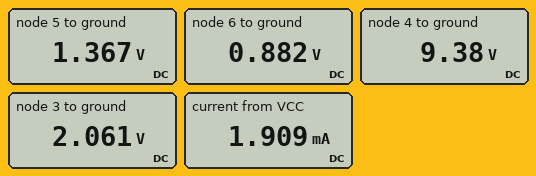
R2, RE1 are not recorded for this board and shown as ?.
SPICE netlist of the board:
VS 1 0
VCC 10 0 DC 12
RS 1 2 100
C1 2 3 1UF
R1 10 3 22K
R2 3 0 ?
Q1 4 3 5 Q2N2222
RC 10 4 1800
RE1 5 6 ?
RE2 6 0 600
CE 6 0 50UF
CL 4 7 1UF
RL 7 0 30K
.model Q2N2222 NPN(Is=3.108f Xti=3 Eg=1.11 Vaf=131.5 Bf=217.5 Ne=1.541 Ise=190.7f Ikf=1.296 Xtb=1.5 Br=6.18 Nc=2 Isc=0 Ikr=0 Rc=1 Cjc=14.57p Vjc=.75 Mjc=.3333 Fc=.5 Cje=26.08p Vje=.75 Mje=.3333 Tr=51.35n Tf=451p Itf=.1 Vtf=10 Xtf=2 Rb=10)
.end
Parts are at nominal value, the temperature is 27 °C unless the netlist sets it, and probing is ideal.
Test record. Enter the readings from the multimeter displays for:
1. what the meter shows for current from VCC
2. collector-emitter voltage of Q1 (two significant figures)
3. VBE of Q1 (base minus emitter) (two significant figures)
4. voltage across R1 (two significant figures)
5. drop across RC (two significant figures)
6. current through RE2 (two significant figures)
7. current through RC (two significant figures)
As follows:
1.909 mA
8.0 V
690 mV
9.9 V
2.6 V
1.5 mA
1.5 mA
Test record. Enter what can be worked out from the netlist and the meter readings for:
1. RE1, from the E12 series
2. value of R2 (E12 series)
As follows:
330 Ω
4.7 kΩ
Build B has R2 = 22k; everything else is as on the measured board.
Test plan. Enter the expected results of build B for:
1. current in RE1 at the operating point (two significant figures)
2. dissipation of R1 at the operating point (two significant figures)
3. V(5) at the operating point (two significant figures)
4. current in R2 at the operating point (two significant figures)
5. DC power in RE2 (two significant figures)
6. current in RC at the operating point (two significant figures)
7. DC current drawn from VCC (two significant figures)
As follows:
4.4 mA
2.3 mW
4.1 V
220 µA
12 mW
4.3 mA
4.7 mA
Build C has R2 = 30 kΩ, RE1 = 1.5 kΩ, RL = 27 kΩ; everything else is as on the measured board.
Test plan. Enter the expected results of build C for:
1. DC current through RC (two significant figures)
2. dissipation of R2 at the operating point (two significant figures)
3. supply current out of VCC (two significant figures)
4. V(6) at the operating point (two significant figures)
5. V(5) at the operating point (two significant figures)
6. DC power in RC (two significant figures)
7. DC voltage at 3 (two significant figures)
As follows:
2.8 mA
1.5 mW
3.0 mA
1.7 V
5.9 V
14 mW
6.6 V
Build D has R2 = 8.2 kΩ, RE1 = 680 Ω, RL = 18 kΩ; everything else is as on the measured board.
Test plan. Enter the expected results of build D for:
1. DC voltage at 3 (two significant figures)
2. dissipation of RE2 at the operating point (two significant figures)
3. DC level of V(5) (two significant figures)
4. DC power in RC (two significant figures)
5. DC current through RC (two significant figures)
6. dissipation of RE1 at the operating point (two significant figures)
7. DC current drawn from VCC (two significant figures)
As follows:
3.2 V
2.2 mW
2.5 V
6.5 mW
1.9 mA
2.5 mW
2.3 mA
